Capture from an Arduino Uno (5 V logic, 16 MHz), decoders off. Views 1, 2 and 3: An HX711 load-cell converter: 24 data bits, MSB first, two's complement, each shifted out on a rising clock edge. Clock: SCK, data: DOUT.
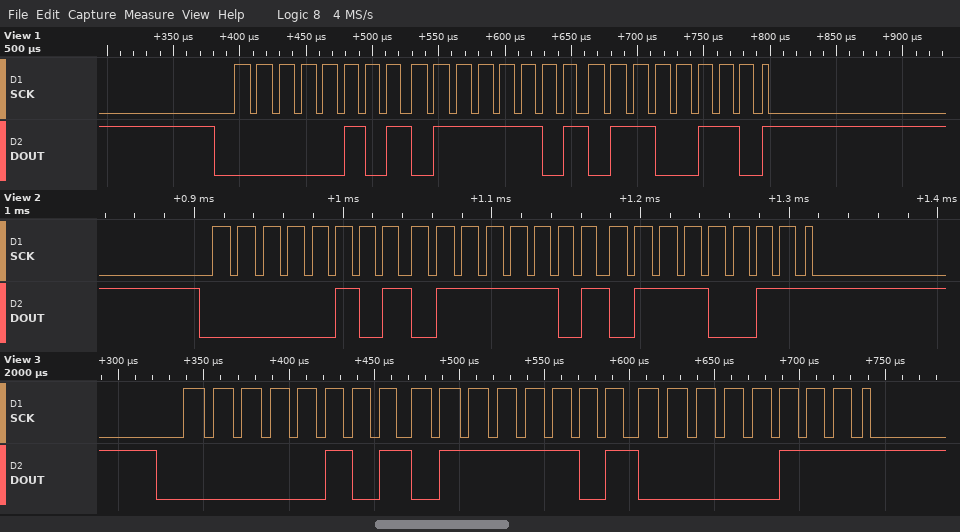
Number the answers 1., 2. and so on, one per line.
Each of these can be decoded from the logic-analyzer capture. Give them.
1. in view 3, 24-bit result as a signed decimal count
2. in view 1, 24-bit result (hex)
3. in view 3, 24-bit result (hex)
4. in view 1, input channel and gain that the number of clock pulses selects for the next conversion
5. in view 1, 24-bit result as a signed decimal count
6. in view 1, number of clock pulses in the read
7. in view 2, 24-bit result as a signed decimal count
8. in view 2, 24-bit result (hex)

1. 359687
2. 0x057D66
3. 0x057D07
4. channel A, gain 128
5. 359782
6. 25
7. 359795
8. 0x057D73
